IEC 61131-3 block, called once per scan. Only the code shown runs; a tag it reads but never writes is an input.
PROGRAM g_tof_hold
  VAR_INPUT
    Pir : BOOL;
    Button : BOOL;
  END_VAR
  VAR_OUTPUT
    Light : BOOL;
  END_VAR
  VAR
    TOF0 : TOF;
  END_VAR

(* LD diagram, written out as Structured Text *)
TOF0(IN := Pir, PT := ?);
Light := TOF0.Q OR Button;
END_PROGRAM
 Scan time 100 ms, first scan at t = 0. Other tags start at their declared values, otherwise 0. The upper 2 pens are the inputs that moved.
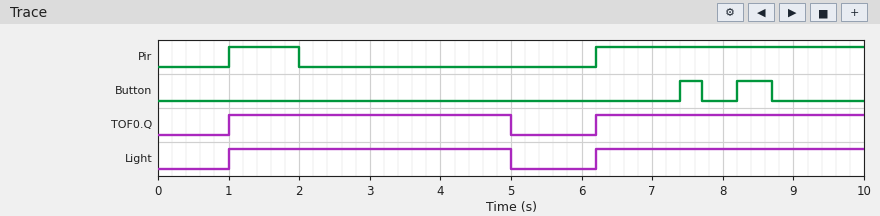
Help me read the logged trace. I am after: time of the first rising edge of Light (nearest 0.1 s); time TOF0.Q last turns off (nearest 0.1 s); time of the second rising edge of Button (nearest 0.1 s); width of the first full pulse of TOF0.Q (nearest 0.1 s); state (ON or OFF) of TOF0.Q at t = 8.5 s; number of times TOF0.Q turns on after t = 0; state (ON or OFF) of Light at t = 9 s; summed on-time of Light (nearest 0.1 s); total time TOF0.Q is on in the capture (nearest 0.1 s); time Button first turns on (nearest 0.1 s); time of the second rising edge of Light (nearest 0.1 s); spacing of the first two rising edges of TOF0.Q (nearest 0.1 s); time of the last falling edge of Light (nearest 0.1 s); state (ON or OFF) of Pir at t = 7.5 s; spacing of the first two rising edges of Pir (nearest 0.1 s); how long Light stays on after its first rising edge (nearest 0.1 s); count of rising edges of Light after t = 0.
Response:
1.0 s
5.0 s
8.2 s
4.0 s
ON
2
ON
7.8 s
7.8 s
7.4 s
6.2 s
5.2 s
5.0 s
ON
5.2 s
4.0 s
2
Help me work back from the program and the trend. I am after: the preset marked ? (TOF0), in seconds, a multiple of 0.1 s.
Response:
3.0 s
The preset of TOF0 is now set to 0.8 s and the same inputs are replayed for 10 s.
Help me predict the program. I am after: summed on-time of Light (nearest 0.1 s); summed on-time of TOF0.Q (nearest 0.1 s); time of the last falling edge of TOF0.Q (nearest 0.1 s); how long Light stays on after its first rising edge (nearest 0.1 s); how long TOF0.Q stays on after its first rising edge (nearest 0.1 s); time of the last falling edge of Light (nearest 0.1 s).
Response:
5.6 s
5.6 s
2.8 s
1.8 s
1.8 s
2.8 s
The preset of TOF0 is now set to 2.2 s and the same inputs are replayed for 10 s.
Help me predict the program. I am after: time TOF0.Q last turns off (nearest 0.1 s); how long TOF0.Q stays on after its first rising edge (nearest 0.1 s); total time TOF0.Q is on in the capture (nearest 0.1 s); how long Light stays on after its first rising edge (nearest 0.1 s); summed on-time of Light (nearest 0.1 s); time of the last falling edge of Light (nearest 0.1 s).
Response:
4.2 s
3.2 s
7.0 s
3.2 s
7.0 s
4.2 s
